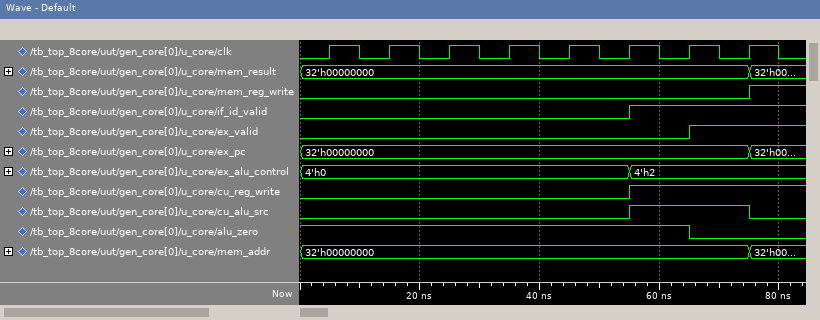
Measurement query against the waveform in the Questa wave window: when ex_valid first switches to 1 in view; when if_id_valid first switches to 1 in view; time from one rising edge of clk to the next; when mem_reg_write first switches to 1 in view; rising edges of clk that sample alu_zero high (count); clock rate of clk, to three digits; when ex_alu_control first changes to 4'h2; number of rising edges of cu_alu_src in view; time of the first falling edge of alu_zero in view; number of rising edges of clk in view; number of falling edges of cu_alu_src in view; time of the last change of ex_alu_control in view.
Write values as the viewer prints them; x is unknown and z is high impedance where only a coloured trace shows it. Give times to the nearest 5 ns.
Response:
65 ns
55 ns
10 ns
75 ns
7
100 MHz
55 ns
1
65 ns
8
1
55 ns
